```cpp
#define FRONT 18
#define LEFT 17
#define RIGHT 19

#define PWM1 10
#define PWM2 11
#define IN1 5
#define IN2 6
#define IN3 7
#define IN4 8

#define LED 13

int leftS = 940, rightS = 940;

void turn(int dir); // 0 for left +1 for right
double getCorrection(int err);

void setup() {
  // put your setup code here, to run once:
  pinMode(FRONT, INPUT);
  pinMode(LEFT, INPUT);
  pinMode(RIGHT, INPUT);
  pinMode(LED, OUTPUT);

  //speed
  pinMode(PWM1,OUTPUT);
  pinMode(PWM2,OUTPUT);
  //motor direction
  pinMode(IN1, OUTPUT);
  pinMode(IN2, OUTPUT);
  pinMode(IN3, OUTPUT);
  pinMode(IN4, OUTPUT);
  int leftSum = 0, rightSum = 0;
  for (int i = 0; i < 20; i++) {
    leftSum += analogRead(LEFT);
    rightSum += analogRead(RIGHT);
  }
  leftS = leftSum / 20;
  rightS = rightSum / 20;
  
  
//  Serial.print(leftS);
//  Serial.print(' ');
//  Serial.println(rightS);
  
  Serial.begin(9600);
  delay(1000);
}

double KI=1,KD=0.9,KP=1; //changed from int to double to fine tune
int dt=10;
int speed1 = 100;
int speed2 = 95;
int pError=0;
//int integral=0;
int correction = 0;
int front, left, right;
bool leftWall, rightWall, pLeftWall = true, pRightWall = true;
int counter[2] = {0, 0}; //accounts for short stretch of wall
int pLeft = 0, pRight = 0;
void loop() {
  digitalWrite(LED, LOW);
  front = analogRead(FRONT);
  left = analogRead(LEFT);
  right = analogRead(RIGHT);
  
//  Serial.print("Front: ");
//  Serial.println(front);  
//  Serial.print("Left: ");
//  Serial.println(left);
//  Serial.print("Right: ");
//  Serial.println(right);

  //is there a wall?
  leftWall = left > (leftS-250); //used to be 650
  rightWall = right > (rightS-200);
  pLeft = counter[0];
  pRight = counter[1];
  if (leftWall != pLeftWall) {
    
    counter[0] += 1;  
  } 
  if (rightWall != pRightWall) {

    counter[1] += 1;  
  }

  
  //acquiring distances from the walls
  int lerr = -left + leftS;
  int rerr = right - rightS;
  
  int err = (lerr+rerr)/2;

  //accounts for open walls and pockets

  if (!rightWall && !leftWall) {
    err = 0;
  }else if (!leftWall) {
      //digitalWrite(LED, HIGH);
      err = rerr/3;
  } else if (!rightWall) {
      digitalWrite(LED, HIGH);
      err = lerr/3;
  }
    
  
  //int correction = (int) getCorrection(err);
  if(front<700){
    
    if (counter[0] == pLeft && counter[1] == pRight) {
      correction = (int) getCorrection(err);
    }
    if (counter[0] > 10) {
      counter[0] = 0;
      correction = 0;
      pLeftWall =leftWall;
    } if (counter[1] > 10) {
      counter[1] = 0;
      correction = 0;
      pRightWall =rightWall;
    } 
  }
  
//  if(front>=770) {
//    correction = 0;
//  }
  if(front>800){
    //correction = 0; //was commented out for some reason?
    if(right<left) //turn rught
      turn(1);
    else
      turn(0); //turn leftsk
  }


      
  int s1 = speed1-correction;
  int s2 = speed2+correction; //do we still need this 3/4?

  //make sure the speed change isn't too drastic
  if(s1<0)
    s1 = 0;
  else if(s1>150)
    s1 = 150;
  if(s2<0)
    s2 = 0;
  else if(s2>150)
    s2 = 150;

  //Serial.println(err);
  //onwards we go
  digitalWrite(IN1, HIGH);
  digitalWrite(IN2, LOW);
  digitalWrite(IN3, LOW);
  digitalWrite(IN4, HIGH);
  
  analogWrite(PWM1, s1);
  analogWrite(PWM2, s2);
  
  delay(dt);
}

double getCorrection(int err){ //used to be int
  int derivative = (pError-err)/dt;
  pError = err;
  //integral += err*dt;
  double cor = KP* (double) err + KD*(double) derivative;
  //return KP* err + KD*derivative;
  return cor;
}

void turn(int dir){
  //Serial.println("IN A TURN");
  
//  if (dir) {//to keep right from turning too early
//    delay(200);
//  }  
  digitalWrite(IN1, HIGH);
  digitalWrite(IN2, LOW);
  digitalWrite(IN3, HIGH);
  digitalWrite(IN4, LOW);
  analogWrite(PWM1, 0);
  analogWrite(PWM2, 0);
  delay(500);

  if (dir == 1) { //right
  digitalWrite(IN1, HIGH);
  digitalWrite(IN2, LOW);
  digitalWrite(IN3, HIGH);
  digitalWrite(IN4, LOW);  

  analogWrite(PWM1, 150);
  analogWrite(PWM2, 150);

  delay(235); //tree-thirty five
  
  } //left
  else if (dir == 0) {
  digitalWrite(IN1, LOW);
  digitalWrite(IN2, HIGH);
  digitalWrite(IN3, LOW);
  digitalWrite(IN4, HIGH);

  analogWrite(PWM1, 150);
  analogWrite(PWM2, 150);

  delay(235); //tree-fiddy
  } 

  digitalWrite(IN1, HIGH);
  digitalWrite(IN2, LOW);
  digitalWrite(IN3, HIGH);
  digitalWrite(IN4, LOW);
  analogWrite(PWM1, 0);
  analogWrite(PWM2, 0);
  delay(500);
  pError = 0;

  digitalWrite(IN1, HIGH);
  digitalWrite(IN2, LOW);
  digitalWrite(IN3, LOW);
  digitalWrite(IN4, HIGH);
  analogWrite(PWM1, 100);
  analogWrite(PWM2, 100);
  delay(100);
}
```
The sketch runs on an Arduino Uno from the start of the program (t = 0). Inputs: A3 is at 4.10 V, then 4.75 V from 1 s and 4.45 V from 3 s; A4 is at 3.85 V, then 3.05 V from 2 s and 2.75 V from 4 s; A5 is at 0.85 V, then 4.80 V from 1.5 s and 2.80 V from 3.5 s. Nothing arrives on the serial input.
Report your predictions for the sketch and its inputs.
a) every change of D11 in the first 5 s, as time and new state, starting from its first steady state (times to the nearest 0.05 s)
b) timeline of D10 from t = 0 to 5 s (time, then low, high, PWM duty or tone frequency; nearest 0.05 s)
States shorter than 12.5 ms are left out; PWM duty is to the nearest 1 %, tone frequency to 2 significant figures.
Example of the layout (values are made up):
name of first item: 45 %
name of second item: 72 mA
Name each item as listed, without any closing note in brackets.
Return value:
every change of D11 in the first 5 s, as time and new state, starting from its first steady state: 0 s low; 1 s PWM 37 %; 2 s PWM 59 %
timeline of D10 from t = 0 to 5 s: 0 s low; 1 s PWM 39 %; 2 s low
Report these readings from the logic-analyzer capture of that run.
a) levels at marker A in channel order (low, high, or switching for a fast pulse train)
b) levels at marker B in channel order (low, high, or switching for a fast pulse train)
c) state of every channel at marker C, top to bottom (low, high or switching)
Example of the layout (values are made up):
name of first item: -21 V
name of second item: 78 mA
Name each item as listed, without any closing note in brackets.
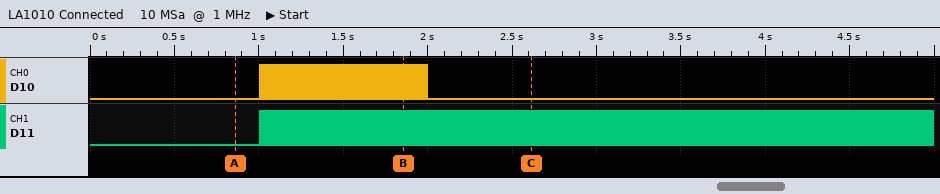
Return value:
levels at marker A in channel order: D10 low, D11 low
levels at marker B in channel order: D10 switching, D11 switching
state of every channel at marker C, top to bottom: D10 low, D11 switching
